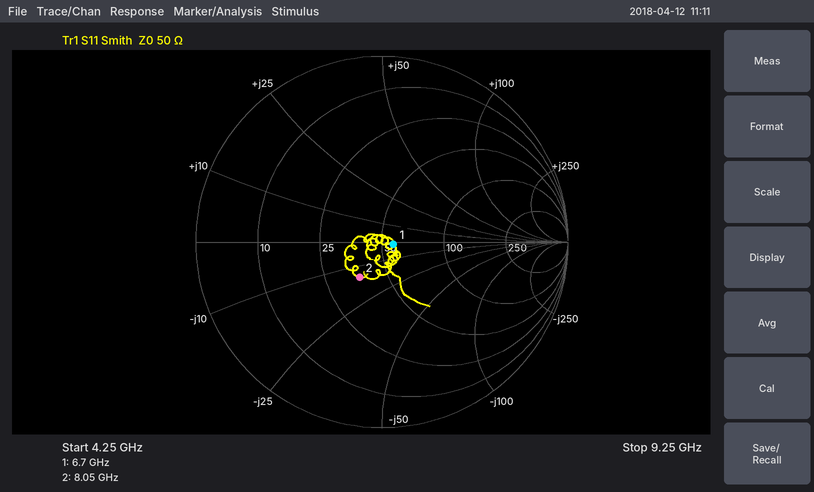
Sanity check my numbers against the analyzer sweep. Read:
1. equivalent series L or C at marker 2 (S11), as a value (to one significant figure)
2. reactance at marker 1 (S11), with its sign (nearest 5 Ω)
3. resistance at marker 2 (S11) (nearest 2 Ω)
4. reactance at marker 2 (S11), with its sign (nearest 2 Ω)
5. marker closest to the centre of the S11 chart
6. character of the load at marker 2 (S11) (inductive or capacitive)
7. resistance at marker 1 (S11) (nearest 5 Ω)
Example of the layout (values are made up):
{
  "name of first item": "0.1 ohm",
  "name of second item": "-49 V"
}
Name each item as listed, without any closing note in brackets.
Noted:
{
  "equivalent series L or C at marker 2 (S11), as a value": "1 pF",
  "reactance at marker 1 (S11), with its sign": "0 Ω",
  "resistance at marker 2 (S11)": "36 Ω",
  "reactance at marker 2 (S11), with its sign": "-14 Ω",
  "marker closest to the centre of the S11 chart": "marker 1",
  "character of the load at marker 2 (S11)": "capacitive",
  "resistance at marker 1 (S11)": "55 Ω"
}
